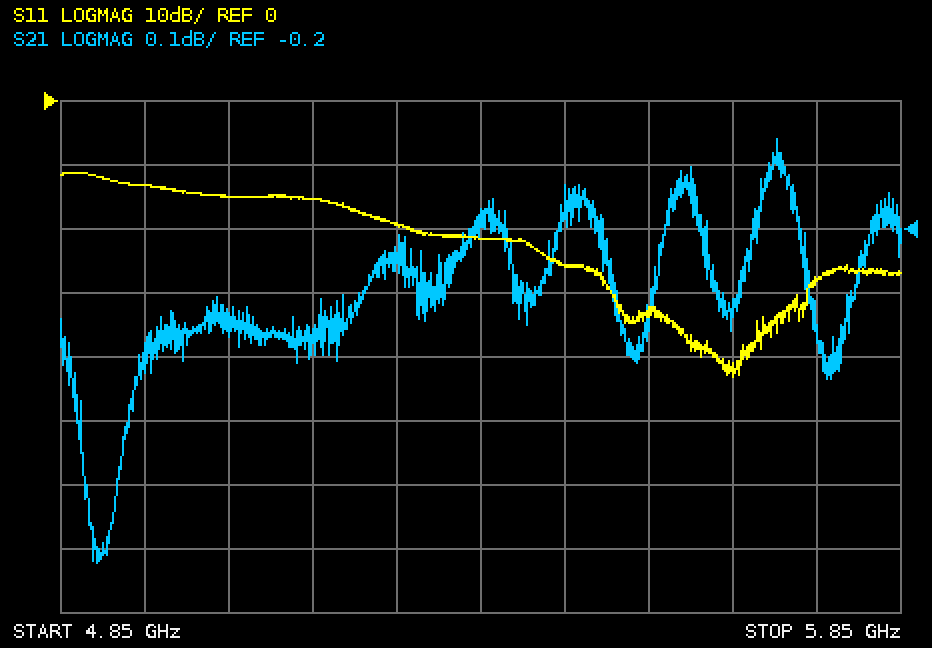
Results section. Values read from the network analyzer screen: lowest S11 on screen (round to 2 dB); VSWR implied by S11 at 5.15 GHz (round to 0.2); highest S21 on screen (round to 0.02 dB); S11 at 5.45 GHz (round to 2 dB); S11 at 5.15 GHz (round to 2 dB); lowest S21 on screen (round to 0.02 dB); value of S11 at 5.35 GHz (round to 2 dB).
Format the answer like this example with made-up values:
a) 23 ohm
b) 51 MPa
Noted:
a) -44 dB
b) 1.4
c) -0.06 dB
d) -26 dB
e) -16 dB
f) -0.72 dB
g) -22 dB
